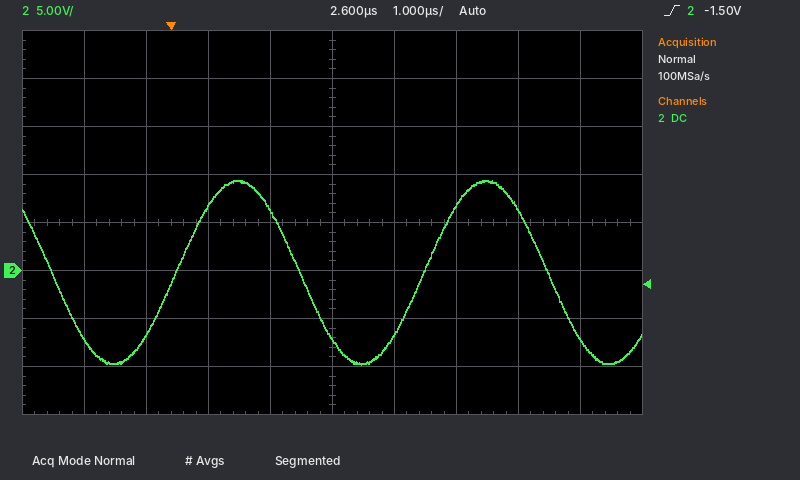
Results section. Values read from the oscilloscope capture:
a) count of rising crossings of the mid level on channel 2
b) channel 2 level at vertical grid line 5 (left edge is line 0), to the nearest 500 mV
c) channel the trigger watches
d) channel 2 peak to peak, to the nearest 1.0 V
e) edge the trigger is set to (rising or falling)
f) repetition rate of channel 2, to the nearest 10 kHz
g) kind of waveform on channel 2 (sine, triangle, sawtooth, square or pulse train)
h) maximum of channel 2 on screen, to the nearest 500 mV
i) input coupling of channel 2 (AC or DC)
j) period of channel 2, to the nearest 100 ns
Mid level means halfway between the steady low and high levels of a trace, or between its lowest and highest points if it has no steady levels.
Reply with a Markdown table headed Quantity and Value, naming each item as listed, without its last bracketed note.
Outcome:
| Quantity | Value |
|---|---|
| count of rising crossings of the mid level on channel 2 | 2 |
| channel 2 level at vertical grid line 5 (left edge is line 0), to the nearest 500 mV | -7.0 V |
| channel the trigger watches | channel 2 |
| channel 2 peak to peak, to the nearest 1.0 V | 19.0 V |
| edge the trigger is set to | rising |
| repetition rate of channel 2, to the nearest 10 kHz | 250 kHz |
| kind of waveform on channel 2 | sine |
| maximum of channel 2 on screen, to the nearest 500 mV | 9.5 V |
| input coupling of channel 2 | DC |
| period of channel 2, to the nearest 100 ns | 4.0 µs |
